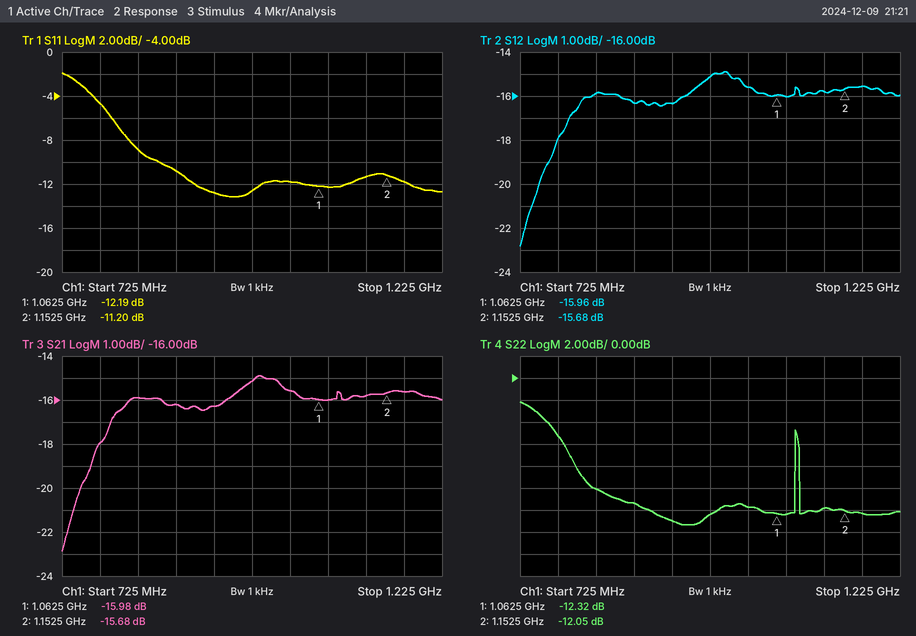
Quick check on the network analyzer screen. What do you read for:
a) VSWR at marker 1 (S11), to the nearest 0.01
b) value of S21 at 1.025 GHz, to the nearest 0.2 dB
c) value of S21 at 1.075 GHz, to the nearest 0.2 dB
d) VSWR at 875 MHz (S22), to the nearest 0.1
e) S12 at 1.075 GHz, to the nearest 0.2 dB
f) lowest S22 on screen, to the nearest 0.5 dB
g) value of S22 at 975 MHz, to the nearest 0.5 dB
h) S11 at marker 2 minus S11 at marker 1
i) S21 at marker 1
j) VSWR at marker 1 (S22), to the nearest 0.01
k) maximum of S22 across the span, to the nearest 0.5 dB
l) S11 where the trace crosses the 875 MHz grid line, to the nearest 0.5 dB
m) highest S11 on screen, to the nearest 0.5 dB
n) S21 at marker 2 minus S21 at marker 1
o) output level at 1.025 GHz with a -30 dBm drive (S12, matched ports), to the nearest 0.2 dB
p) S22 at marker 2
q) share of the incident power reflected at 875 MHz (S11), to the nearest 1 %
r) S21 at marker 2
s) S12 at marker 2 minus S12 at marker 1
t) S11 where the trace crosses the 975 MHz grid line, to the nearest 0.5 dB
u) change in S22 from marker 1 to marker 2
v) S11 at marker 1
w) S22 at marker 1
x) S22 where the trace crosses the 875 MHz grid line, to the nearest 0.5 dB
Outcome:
1.65
-15.6 dB
-16.0 dB
1.7
-16.0 dB
-13.5 dB
-12.5 dB
0.99 dB
-15.98 dB
1.64
-2.0 dB
-11.0 dB
-2.0 dB
0.30 dB
-45.6 dBm
-12.05 dB
8 %
-15.68 dB
0.28 dB
-12.5 dB
0.27 dB
-12.19 dB
-12.32 dB
-11.5 dB
